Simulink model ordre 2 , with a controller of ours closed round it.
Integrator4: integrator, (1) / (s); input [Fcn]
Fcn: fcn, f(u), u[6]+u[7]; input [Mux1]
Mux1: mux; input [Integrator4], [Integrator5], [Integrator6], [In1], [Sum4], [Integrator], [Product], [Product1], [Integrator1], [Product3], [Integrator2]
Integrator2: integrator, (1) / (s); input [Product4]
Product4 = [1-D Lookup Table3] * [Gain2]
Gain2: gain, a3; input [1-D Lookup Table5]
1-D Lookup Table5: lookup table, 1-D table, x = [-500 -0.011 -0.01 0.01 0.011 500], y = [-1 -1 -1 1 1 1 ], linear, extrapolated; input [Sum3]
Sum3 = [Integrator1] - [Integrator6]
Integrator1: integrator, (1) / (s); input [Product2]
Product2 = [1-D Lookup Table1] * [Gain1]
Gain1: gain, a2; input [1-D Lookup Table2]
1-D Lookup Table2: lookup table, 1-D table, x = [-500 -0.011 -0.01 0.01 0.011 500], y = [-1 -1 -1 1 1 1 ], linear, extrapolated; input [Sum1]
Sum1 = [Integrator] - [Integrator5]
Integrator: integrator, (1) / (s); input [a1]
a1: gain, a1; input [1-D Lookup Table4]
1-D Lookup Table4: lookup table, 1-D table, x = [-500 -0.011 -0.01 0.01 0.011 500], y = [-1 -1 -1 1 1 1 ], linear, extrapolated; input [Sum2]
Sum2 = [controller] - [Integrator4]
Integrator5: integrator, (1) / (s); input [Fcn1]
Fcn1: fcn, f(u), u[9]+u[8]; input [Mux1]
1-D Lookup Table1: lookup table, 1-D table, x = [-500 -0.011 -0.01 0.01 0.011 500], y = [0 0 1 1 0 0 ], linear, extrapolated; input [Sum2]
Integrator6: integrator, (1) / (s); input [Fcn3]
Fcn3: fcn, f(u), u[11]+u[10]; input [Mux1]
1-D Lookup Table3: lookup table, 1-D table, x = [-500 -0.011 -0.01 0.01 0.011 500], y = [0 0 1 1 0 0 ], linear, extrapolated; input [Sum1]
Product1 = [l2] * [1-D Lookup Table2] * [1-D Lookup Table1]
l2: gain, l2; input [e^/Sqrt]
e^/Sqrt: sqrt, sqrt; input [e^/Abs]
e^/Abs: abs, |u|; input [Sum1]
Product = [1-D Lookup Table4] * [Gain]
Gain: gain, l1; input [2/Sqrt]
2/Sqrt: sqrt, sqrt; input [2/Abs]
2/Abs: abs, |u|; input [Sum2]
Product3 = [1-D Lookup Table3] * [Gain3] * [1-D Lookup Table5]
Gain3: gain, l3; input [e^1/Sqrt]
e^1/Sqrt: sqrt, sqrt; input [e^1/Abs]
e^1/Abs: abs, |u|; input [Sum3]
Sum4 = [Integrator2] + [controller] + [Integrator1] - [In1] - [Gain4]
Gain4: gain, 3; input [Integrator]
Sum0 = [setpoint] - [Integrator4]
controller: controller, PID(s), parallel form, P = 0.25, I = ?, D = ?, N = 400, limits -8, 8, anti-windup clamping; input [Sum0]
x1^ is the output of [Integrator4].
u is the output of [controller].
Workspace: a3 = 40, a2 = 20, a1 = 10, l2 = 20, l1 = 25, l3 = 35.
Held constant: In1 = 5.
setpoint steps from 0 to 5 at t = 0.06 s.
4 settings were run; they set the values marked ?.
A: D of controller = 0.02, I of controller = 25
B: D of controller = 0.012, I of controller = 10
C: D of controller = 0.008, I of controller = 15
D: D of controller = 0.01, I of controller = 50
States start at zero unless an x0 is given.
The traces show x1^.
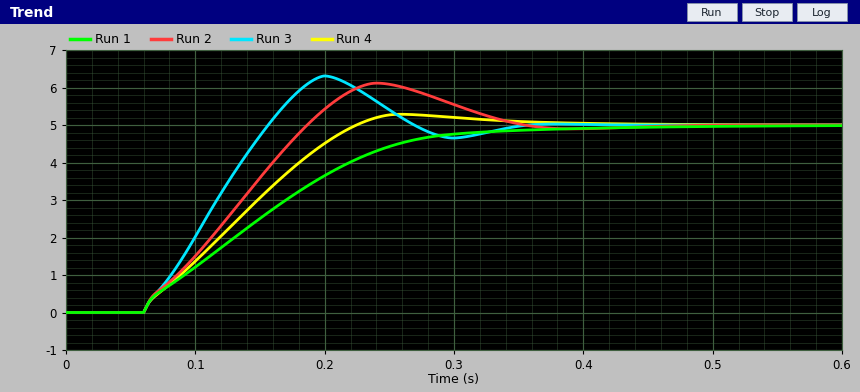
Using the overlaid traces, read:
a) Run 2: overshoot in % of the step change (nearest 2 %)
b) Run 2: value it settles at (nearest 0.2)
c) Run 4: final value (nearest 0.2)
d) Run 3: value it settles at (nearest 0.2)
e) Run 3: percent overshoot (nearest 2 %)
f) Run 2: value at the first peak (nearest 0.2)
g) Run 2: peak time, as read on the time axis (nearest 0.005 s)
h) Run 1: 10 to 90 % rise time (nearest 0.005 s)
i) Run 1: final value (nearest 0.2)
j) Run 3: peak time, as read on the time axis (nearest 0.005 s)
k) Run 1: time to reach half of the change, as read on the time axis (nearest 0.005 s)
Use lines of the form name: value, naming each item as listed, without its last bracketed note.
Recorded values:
Run 2: overshoot in % of the step change: 22 %
Run 2: value it settles at: 5.0
Run 4: final value: 5.0
Run 3: value it settles at: 5.0
Run 3: percent overshoot: 26 %
Run 2: value at the first peak: 6.2
Run 2: peak time, as read on the time axis: 0.240 s
Run 1: 10 to 90 % rise time: 0.185 s
Run 1: final value: 5.0
Run 3: peak time, as read on the time axis: 0.200 s
Run 1: time to reach half of the change, as read on the time axis: 0.150 s
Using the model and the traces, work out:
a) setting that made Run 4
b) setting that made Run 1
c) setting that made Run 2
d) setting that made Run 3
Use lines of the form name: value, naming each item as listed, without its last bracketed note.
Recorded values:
setting that made Run 4: C
setting that made Run 1: B
setting that made Run 2: A
setting that made Run 3: D
